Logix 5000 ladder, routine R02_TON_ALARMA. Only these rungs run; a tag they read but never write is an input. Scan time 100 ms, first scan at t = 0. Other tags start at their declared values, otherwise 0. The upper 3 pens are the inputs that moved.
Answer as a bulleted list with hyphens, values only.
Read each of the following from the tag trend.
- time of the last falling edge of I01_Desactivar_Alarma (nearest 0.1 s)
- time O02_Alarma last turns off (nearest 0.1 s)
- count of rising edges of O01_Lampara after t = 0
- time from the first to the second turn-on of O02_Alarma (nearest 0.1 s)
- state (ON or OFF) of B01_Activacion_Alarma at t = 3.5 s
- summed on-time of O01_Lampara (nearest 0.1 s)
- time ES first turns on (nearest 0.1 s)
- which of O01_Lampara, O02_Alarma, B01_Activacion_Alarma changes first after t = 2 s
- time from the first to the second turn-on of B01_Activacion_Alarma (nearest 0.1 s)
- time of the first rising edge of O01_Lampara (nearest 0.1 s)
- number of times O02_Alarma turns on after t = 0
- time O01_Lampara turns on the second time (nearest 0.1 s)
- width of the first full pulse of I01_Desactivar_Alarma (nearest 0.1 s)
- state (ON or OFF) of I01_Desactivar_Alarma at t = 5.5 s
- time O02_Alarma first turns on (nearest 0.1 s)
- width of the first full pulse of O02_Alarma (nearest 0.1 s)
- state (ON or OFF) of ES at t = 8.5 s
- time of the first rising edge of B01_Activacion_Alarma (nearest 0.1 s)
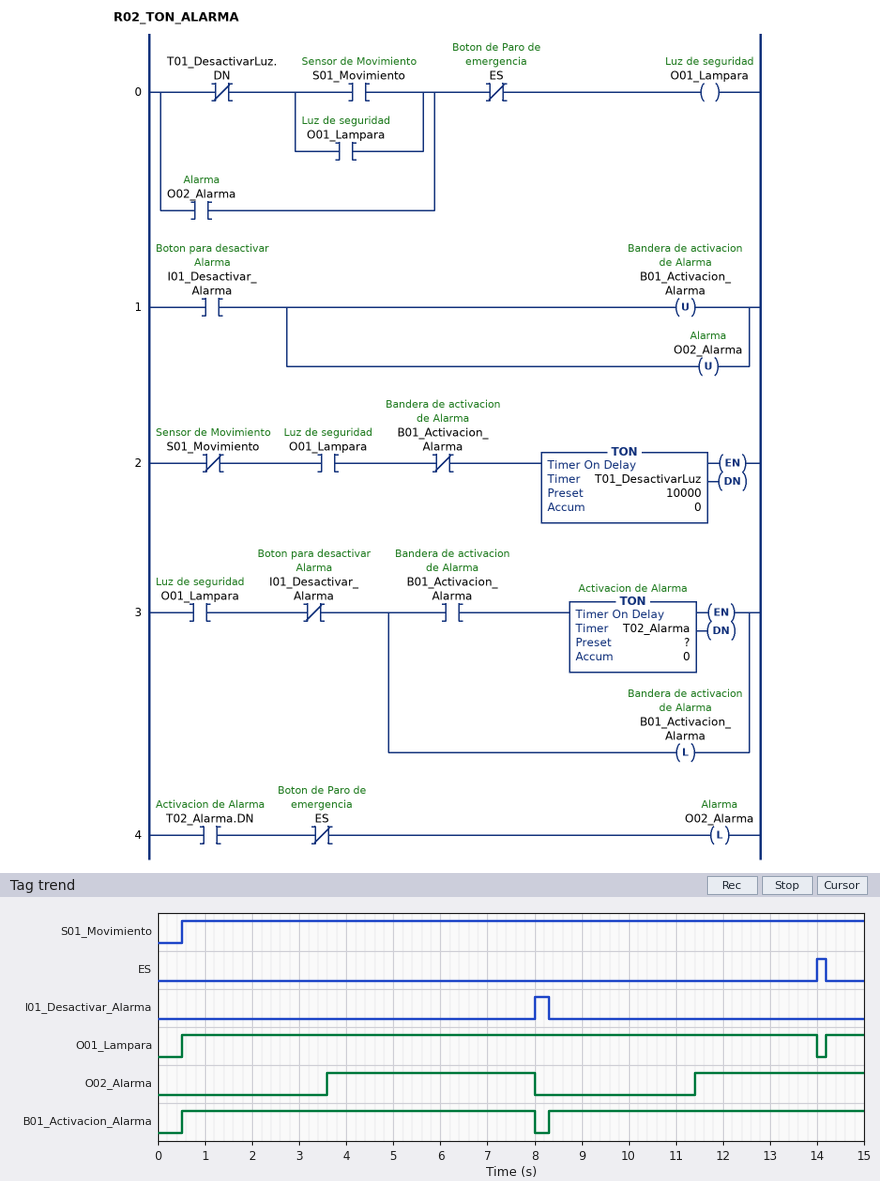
- 8.3 s
- 8.0 s
- 2
- 7.8 s
- ON
- 14.3 s
- 14.0 s
- O02_Alarma
- 7.8 s
- 0.5 s
- 2
- 14.2 s
- 0.3 s
- OFF
- 3.6 s
- 4.4 s
- OFF
- 0.5 s
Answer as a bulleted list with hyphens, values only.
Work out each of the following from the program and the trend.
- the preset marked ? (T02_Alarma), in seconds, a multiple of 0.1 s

- 3.0 s
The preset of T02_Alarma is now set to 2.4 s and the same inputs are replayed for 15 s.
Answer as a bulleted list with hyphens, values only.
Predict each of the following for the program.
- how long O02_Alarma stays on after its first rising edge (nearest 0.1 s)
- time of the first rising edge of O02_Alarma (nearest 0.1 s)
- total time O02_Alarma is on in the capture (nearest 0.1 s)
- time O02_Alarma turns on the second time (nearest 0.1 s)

- 5.0 s
- 3.0 s
- 9.2 s
- 10.8 s
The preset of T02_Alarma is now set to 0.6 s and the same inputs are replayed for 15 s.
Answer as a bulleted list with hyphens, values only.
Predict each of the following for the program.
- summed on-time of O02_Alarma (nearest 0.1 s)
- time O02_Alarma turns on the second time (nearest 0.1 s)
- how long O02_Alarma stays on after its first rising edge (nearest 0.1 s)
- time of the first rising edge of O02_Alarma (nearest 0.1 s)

- 12.8 s
- 9.0 s
- 6.8 s
- 1.2 s
